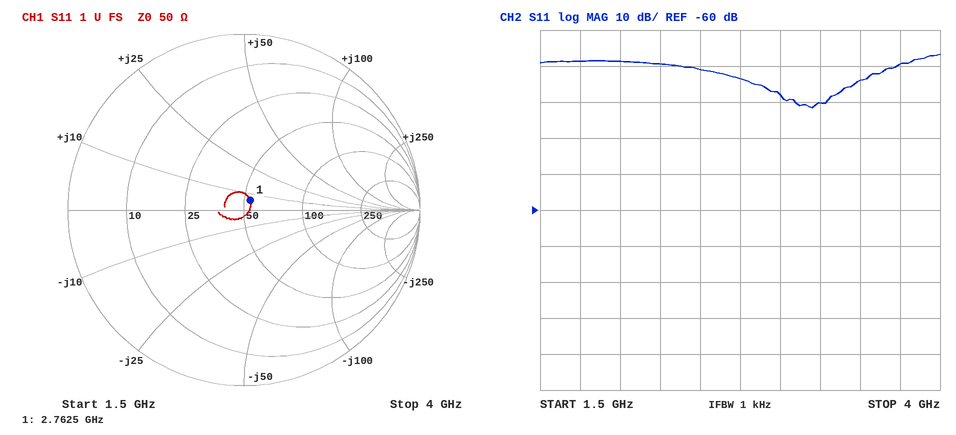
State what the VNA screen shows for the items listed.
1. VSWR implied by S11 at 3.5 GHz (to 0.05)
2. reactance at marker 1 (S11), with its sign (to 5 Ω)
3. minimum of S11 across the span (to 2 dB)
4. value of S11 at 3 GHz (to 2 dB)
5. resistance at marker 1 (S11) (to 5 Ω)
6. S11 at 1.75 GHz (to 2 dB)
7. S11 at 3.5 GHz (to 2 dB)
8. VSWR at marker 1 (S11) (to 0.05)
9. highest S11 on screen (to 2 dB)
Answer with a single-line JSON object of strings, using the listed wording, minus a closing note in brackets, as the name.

{"VSWR implied by S11 at 3.5 GHz": "1.15", "reactance at marker 1 (S11), with its sign": "+5 Ω", "minimum of S11 across the span": "-32 dB", "value of S11 at 3 GHz": "-28 dB", "resistance at marker 1 (S11)": "55 Ω", "S11 at 1.75 GHz": "-18 dB", "S11 at 3.5 GHz": "-24 dB", "VSWR at marker 1 (S11)": "1.15", "highest S11 on screen": "-16 dB"}
